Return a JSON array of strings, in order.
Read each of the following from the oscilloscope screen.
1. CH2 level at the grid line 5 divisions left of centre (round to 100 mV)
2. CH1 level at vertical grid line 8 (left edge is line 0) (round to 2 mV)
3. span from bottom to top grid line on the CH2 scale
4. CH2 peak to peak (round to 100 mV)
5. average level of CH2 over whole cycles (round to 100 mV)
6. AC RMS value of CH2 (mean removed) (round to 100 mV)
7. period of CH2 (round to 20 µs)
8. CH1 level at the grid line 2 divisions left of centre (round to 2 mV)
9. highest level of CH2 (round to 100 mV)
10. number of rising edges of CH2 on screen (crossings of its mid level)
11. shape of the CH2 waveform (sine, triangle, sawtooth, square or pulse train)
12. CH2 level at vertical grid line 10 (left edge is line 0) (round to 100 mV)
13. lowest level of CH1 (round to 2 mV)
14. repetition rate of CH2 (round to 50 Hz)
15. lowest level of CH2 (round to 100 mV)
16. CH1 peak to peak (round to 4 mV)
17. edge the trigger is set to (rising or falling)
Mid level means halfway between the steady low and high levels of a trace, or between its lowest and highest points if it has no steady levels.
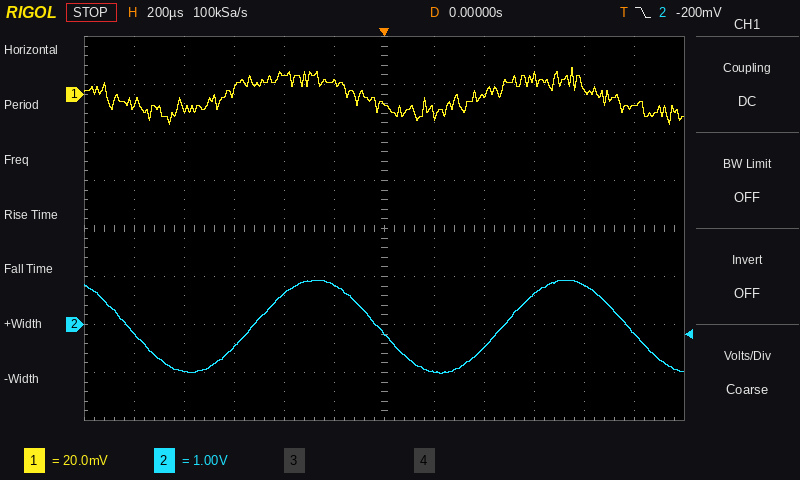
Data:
["-200 mV", "0 mV", "8 V", "1.9 V", "0.0 V", "700 mV", "1.00 ms", "8 mV", "900 mV", "2", "sine", "800 mV", "-12 mV", "1.00 kHz", "-1.0 V", "24 mV", "falling"]
